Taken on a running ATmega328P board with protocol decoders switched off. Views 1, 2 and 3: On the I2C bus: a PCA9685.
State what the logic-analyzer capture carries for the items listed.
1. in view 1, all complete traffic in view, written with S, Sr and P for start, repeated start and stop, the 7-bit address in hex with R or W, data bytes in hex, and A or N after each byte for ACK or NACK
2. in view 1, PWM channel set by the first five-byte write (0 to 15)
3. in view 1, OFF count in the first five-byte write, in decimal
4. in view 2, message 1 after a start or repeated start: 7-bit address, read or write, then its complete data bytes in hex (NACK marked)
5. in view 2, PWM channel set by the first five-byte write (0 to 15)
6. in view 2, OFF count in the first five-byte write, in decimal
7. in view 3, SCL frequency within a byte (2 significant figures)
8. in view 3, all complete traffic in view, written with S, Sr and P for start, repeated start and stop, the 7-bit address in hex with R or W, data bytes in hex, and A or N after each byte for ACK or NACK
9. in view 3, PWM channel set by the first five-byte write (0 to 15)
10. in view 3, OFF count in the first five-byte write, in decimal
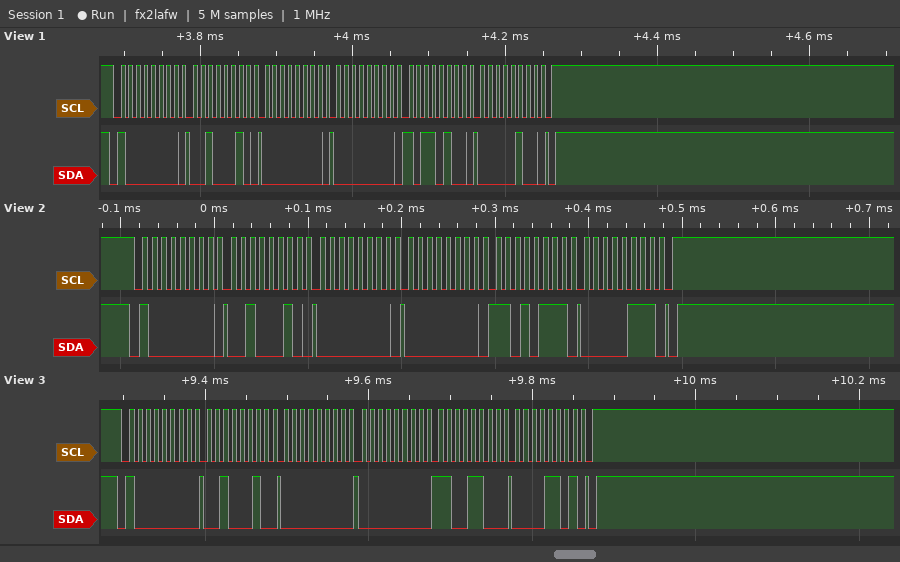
S 40W A 22 A 00 A 00 A B4 A 04 A P
7
1204
0x40 write: 22 00 00 D7 07
7
2007
100 kHz
S 40W A 22 A 00 A 00 A CC A 0D A P
7
3532
